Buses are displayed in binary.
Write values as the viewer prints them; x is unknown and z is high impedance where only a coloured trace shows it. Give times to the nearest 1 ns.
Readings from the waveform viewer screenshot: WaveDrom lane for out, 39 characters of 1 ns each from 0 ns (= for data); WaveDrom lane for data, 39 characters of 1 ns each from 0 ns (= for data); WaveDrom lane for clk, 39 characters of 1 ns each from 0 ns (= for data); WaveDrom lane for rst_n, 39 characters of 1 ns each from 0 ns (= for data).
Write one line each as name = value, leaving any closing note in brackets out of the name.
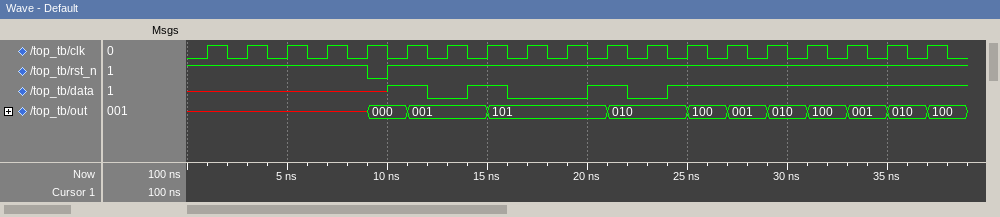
WaveDrom lane for out, 39 characters of 1 ns each from 0 ns = {name: 'out', wave: 'x........=.=...=.....=...=.=.=.=.=.=.=.', data: '000 001 101 010 100 001 010 100 001 010 100'}
WaveDrom lane for data, 39 characters of 1 ns each from 0 ns = {name: 'data', wave: 'x.........1.0.1.0...1.0.1..............'}
WaveDrom lane for clk, 39 characters of 1 ns each from 0 ns = {name: 'clk', wave: '010101010101010101010101010101010101010'}
WaveDrom lane for rst_n, 39 characters of 1 ns each from 0 ns = {name: 'rst_n', wave: '1........01............................'}
